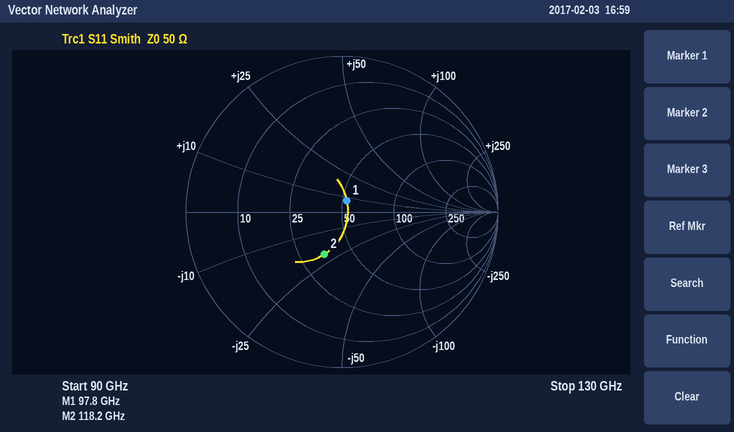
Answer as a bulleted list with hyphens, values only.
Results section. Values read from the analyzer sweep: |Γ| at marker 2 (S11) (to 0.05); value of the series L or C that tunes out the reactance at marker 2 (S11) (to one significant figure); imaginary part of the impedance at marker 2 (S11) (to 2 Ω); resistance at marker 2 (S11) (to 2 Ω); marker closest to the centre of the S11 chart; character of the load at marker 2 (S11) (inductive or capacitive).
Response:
- 0.30
- 30 pH
- -20 Ω
- 34 Ω
- marker 1
- capacitive
